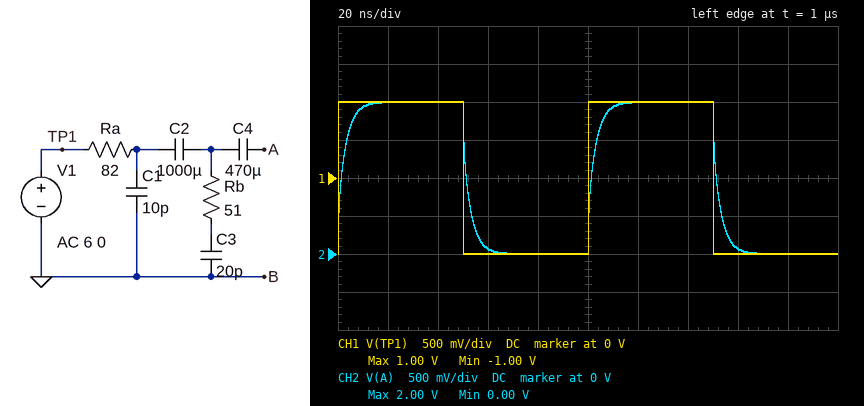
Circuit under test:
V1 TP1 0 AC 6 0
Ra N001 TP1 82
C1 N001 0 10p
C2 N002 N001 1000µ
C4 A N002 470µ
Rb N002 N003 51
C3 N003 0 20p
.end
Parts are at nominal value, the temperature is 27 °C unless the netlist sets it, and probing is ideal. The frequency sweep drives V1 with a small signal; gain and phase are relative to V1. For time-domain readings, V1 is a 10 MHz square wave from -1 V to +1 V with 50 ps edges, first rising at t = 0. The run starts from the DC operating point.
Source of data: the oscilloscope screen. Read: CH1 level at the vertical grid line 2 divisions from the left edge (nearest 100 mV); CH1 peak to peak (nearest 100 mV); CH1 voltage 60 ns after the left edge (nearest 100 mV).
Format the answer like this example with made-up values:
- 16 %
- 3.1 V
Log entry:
- 1.0 V
- 2.0 V
- -1.0 V
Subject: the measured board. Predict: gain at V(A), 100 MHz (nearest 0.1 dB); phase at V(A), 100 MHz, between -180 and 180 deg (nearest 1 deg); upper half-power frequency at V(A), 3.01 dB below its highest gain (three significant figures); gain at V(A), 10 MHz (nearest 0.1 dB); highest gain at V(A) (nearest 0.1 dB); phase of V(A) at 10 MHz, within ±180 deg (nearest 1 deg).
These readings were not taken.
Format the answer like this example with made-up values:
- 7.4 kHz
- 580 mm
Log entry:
- -5.7 dB
- -40 deg
- 54.8 MHz
- -0.2 dB
- 0 dB
- -9 deg
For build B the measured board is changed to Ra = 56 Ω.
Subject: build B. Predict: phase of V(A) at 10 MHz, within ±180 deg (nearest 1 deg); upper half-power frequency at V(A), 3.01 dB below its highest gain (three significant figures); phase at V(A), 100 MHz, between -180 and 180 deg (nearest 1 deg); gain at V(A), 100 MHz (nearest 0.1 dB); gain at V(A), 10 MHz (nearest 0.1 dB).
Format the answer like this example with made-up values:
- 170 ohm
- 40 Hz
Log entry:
- -6 deg
- 78.2 MHz
- -33 deg
- -3.9 dB
- -0.1 dB
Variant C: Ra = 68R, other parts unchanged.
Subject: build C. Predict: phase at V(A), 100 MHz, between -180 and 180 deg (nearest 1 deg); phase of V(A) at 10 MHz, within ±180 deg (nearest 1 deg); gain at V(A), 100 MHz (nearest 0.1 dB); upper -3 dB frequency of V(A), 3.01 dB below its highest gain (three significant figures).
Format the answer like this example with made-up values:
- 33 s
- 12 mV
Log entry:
- -37 deg
- -7 deg
- -4.8 dB
- 65.1 MHz
